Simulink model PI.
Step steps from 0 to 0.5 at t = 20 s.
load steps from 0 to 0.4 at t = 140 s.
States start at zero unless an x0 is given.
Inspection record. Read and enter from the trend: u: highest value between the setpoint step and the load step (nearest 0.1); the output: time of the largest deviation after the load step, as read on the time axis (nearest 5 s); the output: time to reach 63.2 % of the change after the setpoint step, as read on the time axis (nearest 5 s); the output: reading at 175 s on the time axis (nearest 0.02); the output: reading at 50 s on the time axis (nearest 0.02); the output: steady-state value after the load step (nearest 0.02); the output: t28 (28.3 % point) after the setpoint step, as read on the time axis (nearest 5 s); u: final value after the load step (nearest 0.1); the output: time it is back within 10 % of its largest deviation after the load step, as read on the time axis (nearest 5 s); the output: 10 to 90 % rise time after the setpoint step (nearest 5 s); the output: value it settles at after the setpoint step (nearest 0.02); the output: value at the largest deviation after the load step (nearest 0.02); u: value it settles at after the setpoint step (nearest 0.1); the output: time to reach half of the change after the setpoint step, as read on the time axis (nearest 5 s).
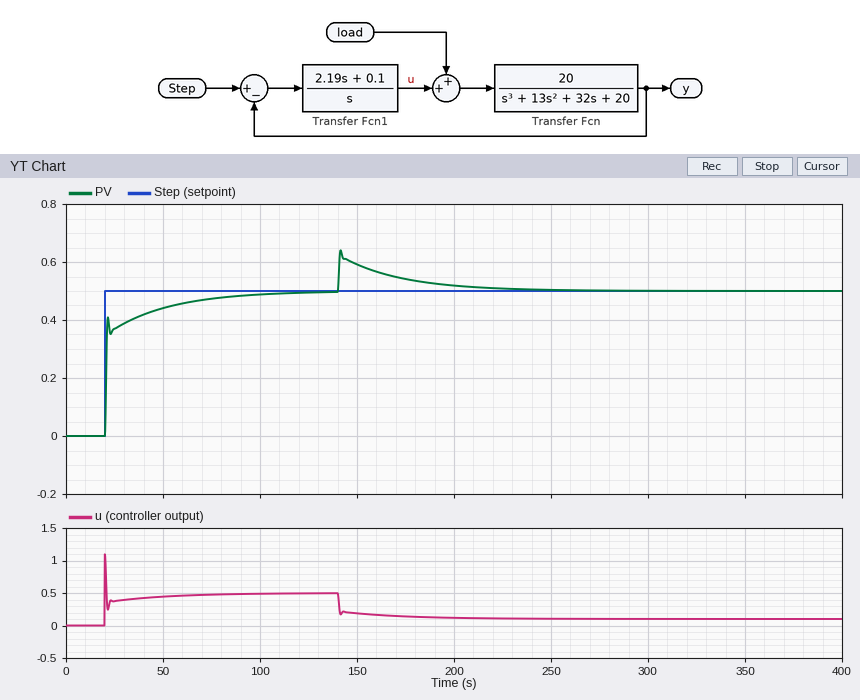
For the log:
1.1
140 s
20 s
0.54
0.44
0.50
20 s
0.1
210 s
35 s
0.50
0.64
0.5
20 s
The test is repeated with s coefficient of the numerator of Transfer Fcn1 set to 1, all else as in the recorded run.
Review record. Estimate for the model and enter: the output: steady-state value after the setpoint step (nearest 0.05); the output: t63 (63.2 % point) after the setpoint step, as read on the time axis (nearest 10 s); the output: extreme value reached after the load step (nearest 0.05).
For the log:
0.50
30 s
0.70
